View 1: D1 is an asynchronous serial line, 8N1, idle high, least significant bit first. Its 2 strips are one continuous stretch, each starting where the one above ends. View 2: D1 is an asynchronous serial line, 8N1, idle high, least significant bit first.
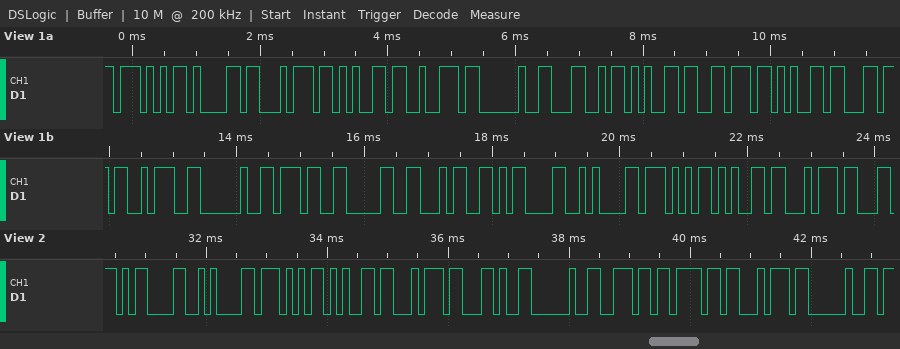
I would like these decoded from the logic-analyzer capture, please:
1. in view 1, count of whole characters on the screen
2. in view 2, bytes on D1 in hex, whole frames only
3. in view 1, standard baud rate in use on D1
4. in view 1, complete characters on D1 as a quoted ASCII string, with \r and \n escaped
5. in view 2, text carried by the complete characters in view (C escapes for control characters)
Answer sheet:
21
0x0D 0x0A 0x57 0x65 0x74 0x2C 0x20 0x6E 0x6F 0x74 0x20
9600 baud
"Water Level: 704\r\nWet"
"\r\nWet, not "
